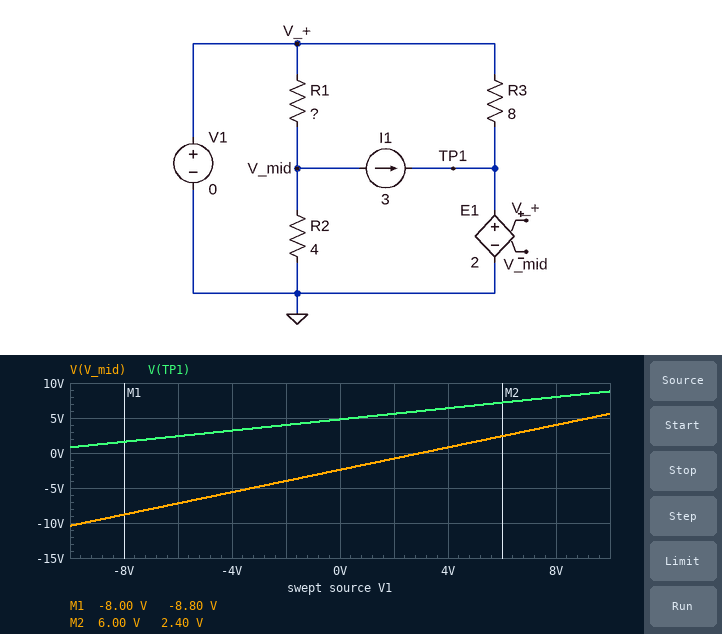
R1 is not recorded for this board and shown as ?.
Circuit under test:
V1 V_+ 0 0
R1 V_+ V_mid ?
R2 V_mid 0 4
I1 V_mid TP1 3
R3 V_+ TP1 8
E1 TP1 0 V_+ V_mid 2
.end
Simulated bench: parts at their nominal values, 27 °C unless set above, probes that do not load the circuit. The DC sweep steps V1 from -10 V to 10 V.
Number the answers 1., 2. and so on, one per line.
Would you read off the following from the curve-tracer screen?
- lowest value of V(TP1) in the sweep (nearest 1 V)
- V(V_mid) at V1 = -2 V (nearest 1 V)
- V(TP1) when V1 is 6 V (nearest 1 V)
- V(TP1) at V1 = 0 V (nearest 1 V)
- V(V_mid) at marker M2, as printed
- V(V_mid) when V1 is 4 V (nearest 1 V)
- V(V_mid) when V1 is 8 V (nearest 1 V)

1. 1 V
2. -4 V
3. 7 V
4. 5 V
5. 2.40 V
6. 1 V
7. 4 V
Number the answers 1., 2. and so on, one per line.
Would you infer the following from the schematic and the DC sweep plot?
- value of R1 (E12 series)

1. 1 Ω
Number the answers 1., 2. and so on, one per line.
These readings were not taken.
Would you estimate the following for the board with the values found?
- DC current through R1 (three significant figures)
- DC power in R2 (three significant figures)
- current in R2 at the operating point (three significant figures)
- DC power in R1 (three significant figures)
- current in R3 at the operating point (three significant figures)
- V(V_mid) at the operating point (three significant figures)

1. 2.40 A
2. 1.44 W
3. 600 mA
4. 5.76 W
5. 600 mA
6. -2.40 V
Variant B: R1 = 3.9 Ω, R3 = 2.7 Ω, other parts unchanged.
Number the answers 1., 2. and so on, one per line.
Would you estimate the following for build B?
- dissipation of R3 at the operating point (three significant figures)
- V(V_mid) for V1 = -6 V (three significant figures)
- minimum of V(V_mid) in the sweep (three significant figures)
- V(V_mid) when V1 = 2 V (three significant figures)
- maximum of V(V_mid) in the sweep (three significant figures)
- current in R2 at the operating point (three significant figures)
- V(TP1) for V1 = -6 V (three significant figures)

1. 52.0 W
2. -8.96 V
3. -11.0 V
4. -4.91 V
5. -861 mV
6. 1.48 A
7. 5.92 V
